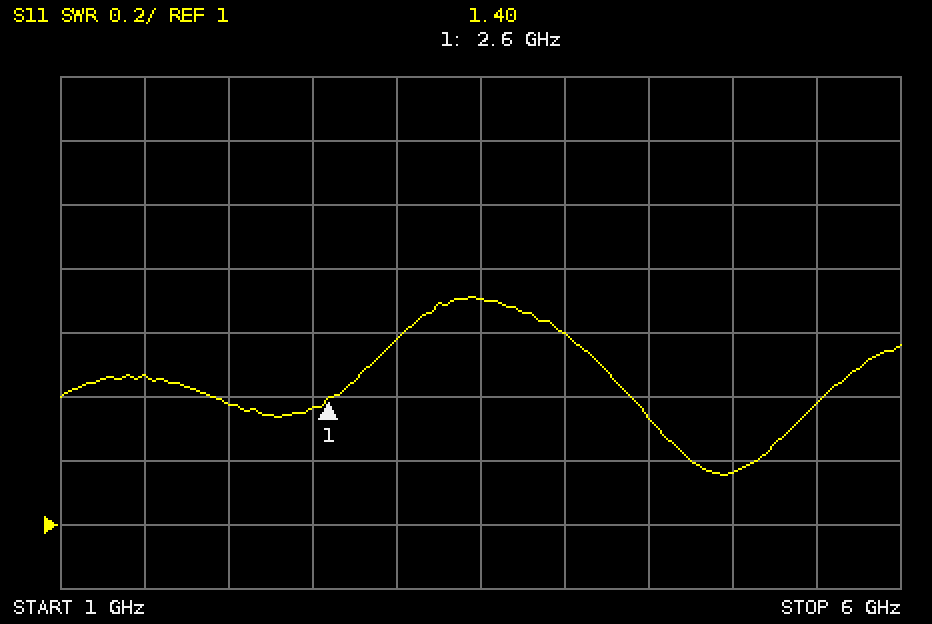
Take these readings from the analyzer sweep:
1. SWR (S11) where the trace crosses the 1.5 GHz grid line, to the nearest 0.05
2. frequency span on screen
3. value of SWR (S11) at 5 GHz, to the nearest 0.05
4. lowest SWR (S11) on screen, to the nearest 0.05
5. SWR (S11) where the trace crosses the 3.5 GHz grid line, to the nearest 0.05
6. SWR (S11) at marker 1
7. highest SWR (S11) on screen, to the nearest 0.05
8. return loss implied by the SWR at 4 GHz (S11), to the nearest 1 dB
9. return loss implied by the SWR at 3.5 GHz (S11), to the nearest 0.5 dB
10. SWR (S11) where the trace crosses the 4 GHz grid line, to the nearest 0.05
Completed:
1.45
5 GHz
1.15
1.15
1.70
1.40
1.70
13 dB
11.5 dB
1.60
